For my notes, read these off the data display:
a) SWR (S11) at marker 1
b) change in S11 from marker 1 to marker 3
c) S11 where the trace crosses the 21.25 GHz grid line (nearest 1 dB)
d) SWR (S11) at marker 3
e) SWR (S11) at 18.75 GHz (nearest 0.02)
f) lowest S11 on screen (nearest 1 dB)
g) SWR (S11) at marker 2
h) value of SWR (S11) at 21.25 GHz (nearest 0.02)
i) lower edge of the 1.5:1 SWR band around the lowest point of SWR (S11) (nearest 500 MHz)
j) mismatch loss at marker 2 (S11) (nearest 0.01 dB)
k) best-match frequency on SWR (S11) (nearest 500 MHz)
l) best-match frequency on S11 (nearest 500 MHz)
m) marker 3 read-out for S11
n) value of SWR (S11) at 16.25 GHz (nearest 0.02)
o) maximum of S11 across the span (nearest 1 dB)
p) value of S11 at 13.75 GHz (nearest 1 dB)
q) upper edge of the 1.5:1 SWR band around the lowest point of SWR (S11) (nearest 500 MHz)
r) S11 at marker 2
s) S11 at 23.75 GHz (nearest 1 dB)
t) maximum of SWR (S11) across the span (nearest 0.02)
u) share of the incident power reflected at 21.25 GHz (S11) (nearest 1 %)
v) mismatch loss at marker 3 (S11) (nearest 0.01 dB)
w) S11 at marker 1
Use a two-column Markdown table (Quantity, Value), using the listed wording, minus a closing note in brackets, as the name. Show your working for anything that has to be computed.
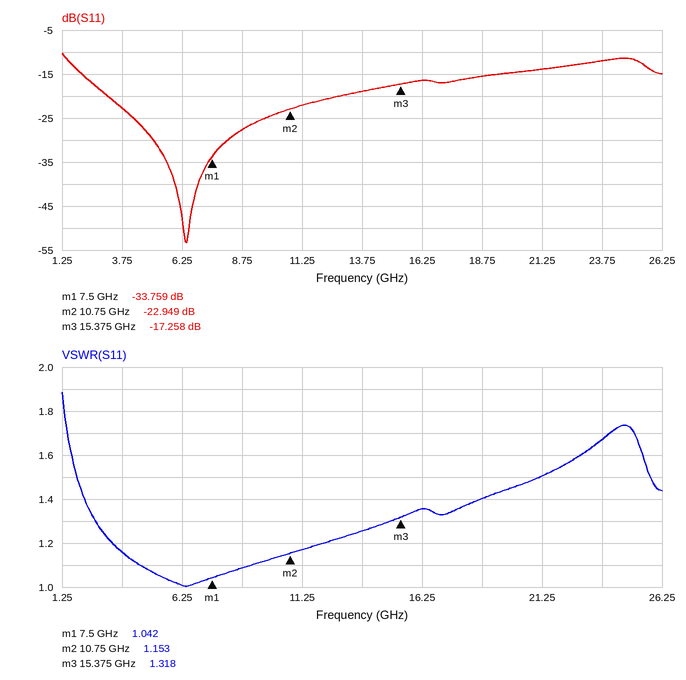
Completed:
| Quantity | Value |
|---|---|
| SWR (S11) at marker 1 | 1.042 |
| change in S11 from marker 1 to marker 3 | -17.258 − (-33.759) = 16.501 dB |
| S11 where the trace crosses the 21.25 GHz grid line | -14 dB |
| SWR (S11) at marker 3 | 1.318 |
| SWR (S11) at 18.75 GHz | 1.40 |
| lowest S11 on screen | -53 dB |
| SWR (S11) at marker 2 | 1.153 |
| value of SWR (S11) at 21.25 GHz | 1.50 |
| lower edge of the 1.5:1 SWR band around the lowest point of SWR (S11) | 2.0 GHz |
| mismatch loss at marker 2 (S11) | −10 log10(1 − 10^(-22.949/10)) ≈ 0.02 dB |
| best-match frequency on SWR (S11) | 6.5 GHz |
| best-match frequency on S11 | 6.5 GHz |
| marker 3 read-out for S11 | -17.258 dB |
| value of SWR (S11) at 16.25 GHz | 1.36 |
| maximum of S11 across the span | -10 dB |
| value of S11 at 13.75 GHz | -19 dB |
| upper edge of the 1.5:1 SWR band around the lowest point of SWR (S11) | 21.0 GHz |
| S11 at marker 2 | -22.949 dB |
| S11 at 23.75 GHz | -12 dB |
| maximum of SWR (S11) across the span | 1.88 |
| share of the incident power reflected at 21.25 GHz (S11) | 10^(-14/10) ≈ 4 % |
| mismatch loss at marker 3 (S11) | −10 log10(1 − 10^(-17.258/10)) ≈ 0.08 dB |
| S11 at marker 1 | -33.759 dB |
